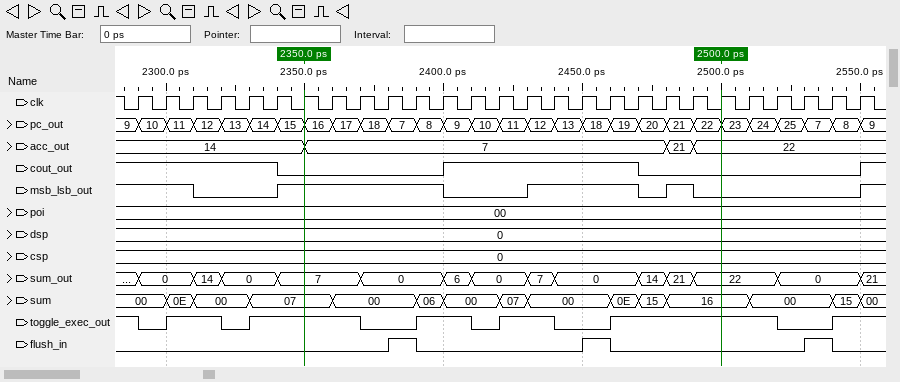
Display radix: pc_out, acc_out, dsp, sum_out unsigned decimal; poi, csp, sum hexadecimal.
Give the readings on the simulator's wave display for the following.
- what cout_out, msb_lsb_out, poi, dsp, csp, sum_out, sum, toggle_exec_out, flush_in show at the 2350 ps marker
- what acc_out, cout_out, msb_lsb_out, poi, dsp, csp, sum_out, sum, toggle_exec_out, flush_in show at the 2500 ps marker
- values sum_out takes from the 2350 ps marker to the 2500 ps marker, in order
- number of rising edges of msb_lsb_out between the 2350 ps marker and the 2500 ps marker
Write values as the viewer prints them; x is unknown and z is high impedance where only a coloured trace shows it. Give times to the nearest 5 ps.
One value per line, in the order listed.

cout_out=0, msb_lsb_out=1, poi=00, dsp=0, csp=0, sum_out=7, sum=07, toggle_exec_out=1, flush_in=0
acc_out=22, cout_out=0, msb_lsb_out=0, poi=00, dsp=0, csp=0, sum_out=22, sum=16, toggle_exec_out=1, flush_in=0
7, 0, 6, 0, 7, 0, 14, 21, 22
2
